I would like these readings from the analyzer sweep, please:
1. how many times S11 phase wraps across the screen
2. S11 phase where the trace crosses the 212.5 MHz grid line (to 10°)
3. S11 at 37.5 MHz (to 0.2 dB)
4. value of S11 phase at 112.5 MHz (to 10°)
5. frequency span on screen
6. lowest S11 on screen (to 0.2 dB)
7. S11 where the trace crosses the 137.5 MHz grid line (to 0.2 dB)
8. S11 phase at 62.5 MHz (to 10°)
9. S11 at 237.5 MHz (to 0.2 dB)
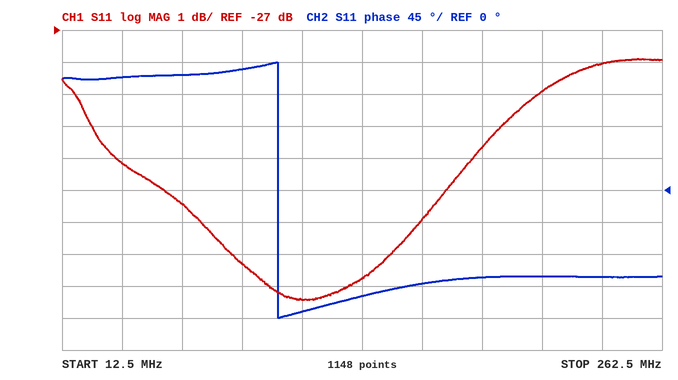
1
-120°
-31.2 dB
-170°
250 MHz
-35.4 dB
-34.8 dB
160°
-28.0 dB
